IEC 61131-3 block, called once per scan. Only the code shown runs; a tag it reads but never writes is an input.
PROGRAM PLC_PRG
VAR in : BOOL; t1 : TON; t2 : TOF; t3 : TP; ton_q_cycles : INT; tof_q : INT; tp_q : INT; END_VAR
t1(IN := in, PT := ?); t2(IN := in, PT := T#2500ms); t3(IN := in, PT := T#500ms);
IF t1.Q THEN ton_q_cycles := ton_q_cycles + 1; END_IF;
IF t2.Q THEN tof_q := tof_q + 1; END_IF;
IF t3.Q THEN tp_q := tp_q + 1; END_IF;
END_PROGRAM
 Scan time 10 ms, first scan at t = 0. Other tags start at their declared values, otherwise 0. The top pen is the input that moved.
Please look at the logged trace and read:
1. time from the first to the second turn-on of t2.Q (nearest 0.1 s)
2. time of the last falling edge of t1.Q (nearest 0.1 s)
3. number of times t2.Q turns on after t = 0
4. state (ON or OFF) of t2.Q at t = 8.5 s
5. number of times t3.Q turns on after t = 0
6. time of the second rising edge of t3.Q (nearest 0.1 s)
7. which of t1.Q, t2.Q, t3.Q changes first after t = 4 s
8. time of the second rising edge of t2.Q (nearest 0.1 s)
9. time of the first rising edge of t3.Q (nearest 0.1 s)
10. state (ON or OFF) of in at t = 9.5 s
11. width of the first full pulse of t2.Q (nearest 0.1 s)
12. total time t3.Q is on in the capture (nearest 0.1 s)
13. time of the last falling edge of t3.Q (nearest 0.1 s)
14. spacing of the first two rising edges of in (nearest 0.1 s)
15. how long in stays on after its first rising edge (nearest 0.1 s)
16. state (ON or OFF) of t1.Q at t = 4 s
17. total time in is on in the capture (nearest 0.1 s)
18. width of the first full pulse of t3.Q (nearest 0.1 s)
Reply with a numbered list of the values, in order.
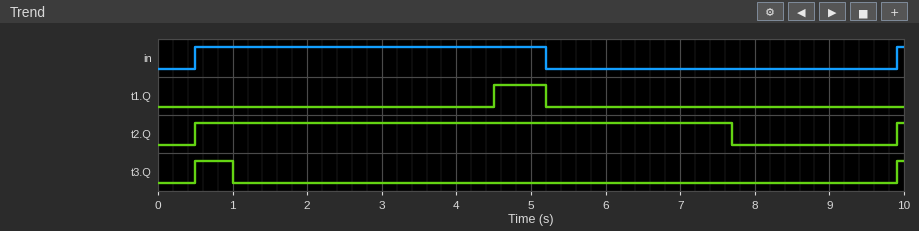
1. 9.4 s
2. 5.2 s
3. 2
4. OFF
5. 2
6. 9.9 s
7. t1.Q
8. 9.9 s
9. 0.5 s
10. OFF
11. 7.2 s
12. 0.6 s
13. 1.0 s
14. 9.4 s
15. 4.7 s
16. OFF
17. 4.8 s
18. 0.5 s
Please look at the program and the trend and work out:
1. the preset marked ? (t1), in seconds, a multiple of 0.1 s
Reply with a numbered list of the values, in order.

1. 4.0 s
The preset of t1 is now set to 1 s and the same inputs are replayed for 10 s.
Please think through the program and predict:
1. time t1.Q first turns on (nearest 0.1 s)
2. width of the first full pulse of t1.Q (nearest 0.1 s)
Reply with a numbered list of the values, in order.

1. 1.5 s
2. 3.7 s
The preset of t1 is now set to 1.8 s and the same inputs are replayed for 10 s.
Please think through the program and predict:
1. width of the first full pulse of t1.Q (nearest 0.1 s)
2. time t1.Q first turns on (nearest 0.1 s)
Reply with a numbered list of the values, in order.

1. 2.9 s
2. 2.3 s
